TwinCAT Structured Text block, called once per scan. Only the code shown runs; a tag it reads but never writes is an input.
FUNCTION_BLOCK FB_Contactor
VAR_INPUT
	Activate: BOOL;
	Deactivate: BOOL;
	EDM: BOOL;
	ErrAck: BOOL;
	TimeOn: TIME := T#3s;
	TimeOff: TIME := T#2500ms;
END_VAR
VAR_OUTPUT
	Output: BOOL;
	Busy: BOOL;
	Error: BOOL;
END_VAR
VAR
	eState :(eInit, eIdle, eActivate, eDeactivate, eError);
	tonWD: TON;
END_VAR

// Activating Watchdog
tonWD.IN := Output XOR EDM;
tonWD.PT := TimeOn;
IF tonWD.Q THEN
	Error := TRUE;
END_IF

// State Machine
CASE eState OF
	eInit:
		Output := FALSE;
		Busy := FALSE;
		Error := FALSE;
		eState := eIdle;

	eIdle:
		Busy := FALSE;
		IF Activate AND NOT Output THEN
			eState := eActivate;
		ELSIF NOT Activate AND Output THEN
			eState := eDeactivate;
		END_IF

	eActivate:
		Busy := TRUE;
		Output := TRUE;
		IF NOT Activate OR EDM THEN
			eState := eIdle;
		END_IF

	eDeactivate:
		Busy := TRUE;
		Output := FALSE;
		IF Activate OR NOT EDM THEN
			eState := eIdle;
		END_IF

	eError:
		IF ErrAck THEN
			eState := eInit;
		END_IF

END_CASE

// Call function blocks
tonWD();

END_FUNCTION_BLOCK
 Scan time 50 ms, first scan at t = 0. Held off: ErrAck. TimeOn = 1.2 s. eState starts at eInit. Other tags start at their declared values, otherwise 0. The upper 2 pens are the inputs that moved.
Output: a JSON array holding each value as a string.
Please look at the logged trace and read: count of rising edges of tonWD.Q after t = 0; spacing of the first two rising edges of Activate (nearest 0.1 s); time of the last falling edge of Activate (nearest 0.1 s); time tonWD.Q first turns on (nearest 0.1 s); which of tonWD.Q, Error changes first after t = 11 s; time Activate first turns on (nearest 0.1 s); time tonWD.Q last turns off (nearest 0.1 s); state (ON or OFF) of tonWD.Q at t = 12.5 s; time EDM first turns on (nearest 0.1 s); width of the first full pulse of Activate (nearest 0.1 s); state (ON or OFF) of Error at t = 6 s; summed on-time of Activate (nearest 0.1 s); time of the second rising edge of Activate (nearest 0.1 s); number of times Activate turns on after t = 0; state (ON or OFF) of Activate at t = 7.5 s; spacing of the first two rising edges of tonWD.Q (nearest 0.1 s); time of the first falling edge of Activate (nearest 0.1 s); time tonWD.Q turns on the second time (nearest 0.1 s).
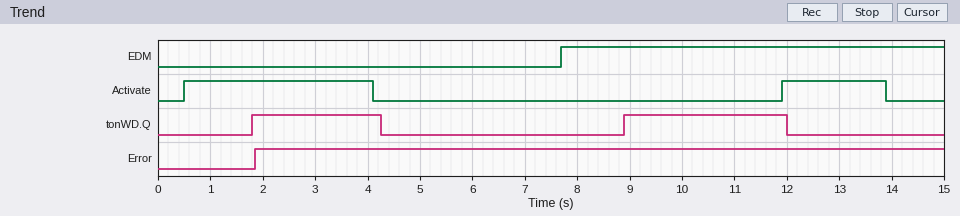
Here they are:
["2", "11.4 s", "13.9 s", "1.8 s", "tonWD.Q", "0.5 s", "12.0 s", "OFF", "7.7 s", "3.6 s", "ON", "5.6 s", "11.9 s", "2", "OFF", "7.1 s", "4.1 s", "8.9 s"]
